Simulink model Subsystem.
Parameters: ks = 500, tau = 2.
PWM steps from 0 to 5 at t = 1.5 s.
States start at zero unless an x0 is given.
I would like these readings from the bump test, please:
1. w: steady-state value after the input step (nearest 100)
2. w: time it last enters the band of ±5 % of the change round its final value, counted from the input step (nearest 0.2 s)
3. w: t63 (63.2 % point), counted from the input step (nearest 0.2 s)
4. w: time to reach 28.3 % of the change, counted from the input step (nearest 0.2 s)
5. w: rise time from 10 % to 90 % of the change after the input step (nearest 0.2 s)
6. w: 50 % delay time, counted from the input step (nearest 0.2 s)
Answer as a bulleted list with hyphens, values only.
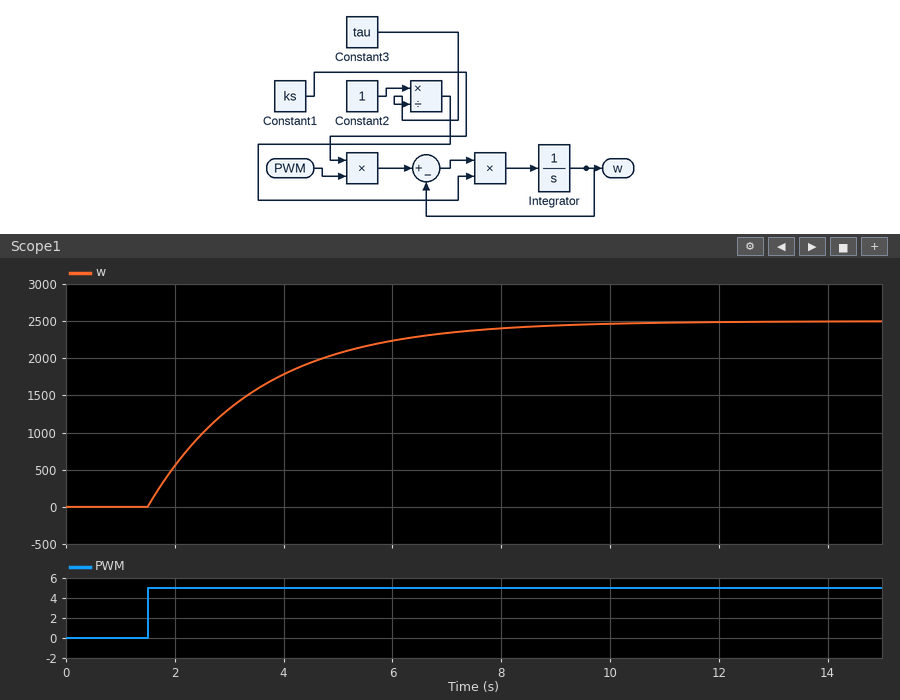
- 2500
- 6.0 s
- 2.0 s
- 0.6 s
- 4.4 s
- 1.4 s
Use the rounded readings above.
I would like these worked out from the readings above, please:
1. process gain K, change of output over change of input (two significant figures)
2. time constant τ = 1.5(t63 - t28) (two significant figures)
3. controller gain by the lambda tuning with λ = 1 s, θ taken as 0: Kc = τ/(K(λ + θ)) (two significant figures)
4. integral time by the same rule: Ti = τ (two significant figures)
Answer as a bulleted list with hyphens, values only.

- 500
- 2.1 s
- 0.0042
- 2.1 s
